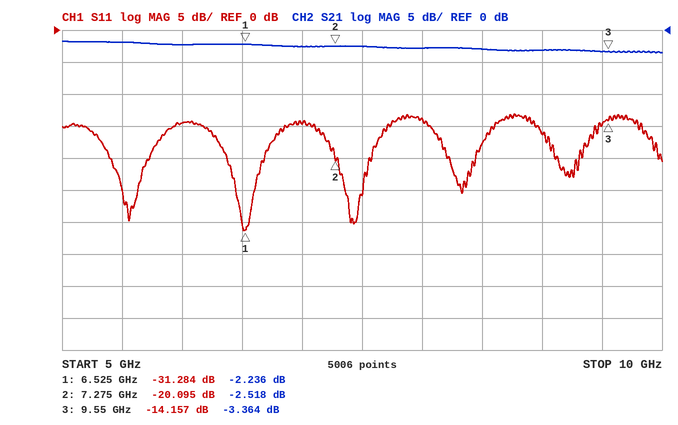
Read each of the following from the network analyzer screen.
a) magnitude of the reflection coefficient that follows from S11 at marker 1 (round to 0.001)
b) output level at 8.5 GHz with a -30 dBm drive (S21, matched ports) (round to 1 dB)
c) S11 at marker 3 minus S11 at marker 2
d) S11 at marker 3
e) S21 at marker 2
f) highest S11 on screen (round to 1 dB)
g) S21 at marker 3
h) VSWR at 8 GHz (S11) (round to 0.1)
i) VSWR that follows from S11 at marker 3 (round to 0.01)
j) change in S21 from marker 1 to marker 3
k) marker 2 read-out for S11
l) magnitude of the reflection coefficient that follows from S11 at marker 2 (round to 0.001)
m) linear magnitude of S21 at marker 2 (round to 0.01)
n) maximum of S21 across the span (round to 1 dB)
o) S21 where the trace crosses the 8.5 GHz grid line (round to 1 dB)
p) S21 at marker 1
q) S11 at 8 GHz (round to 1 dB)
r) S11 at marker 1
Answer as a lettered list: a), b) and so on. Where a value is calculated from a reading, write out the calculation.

a) 10^(-31.284/20) ≈ 0.027
b) -30 dBm + (-3 dB) = -33 dBm
c) -14.157 − (-20.095) = 5.938 dB
d) -14.157 dB
e) -2.518 dB
f) -13 dB
g) -3.364 dB
h) |Γ| = 10^(-14/20) = 0.1995; VSWR = (1 + 0.1995)/(1 − 0.1995) ≈ 1.5
i) (1 + 0.1960)/(1 − 0.1960) ≈ 1.49
j) -3.364 − (-2.236) = -1.128 dB
k) -20.095 dB
l) 10^(-20.095/20) ≈ 0.099
m) 10^(-2.518/20) ≈ 0.75
n) -2 dB
o) -3 dB
p) -2.236 dB
q) -14 dB
r) -31.284 dB
